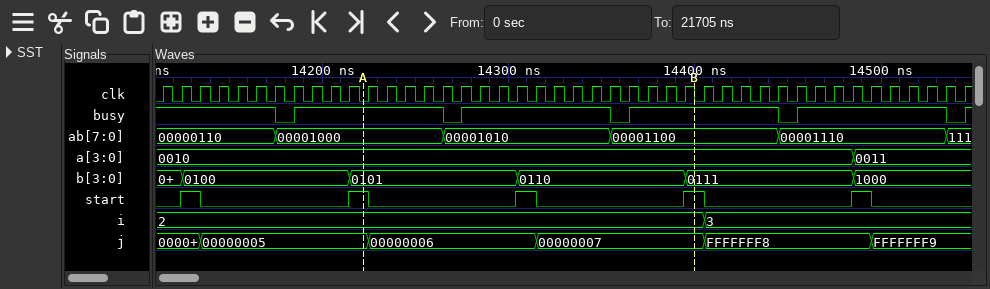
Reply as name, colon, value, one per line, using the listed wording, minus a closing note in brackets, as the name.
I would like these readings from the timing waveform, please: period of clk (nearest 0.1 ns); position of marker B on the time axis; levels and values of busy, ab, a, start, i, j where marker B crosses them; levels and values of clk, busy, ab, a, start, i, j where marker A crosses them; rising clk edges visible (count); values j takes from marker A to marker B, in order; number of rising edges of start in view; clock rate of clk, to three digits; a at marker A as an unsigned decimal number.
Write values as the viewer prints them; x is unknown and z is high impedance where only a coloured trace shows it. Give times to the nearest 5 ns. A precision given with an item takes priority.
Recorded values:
period of clk: 10 ns
position of marker B on the time axis: 14400 ns
levels and values of busy, ab, a, start, i, j where marker B crosses them: busy=1, ab=00001100, a=0010, start=1, i=2, j=00000007
levels and values of clk, busy, ab, a, start, i, j where marker A crosses them: clk=0, busy=1, ab=00001000, a=0010, start=1, i=2, j=00000005
rising clk edges visible: 44
values j takes from marker A to marker B, in order: 00000005, 00000006, 00000007
number of rising edges of start in view: 5
clock rate of clk, to three digits: 100 MHz
a at marker A as an unsigned decimal number: 2
